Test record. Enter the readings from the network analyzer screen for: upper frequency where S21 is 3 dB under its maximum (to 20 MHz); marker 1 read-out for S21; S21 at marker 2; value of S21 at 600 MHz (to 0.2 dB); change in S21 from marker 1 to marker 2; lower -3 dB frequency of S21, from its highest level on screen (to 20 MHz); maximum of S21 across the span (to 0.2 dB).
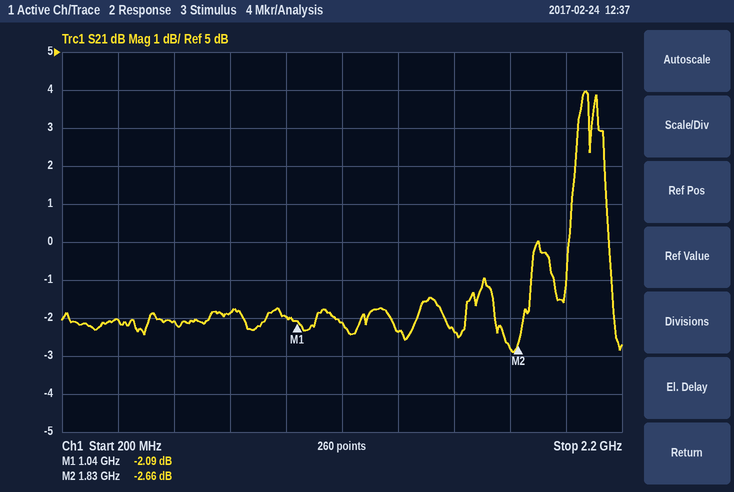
2.14 GHz
-2.09 dB
-2.66 dB
-2.0 dB
-0.57 dB
2.02 GHz
4.0 dB
